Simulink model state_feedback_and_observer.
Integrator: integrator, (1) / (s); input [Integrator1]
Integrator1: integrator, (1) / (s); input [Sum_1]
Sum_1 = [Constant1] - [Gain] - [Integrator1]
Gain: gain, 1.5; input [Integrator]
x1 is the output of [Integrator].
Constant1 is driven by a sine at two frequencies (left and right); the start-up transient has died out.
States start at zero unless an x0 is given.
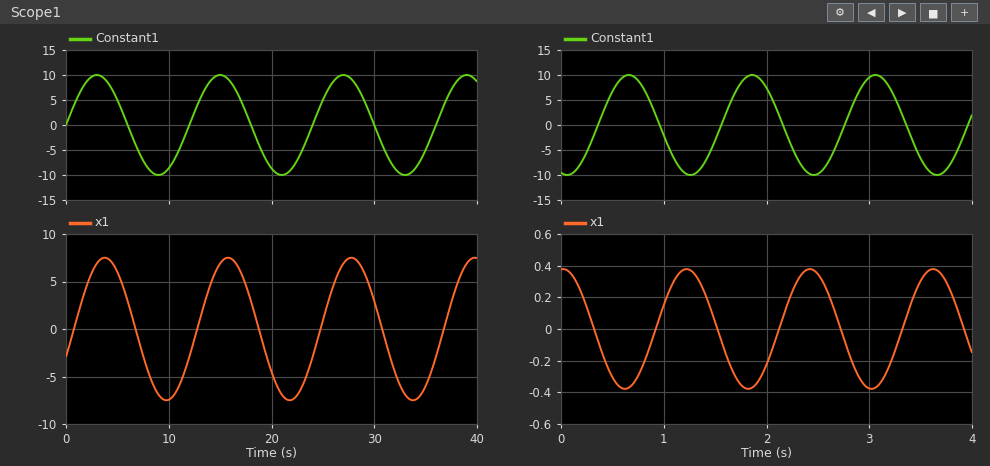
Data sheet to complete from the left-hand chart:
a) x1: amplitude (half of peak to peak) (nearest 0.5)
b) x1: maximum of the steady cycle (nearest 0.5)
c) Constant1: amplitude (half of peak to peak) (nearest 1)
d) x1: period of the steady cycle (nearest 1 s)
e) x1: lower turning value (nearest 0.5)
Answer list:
7.5
7.5
10
12 s
-7.5
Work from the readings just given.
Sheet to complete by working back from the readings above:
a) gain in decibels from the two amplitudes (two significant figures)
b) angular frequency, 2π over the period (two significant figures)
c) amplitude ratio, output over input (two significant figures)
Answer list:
-2.5 dB
0.52 rad/s
0.75
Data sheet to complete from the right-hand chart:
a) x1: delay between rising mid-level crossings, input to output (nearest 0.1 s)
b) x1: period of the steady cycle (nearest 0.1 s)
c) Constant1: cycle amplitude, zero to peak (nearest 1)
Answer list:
0.6 s
1.2 s
10
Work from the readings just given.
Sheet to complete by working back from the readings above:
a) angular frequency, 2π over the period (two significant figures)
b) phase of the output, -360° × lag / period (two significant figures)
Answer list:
5.2 rad/s
-180°
